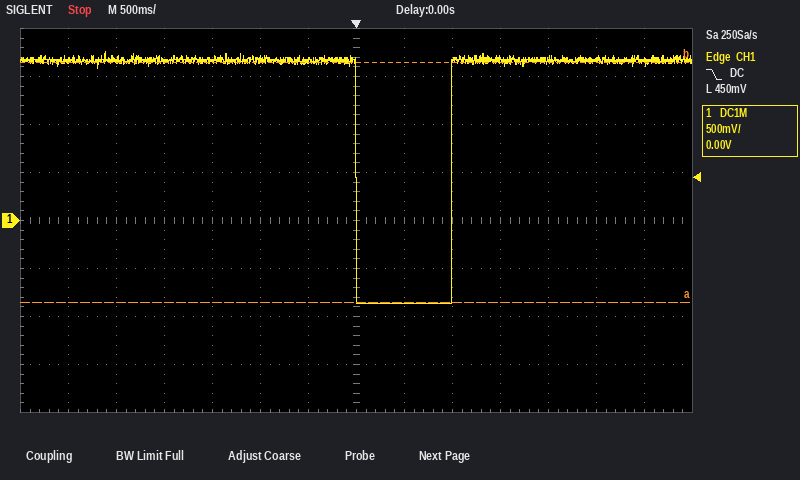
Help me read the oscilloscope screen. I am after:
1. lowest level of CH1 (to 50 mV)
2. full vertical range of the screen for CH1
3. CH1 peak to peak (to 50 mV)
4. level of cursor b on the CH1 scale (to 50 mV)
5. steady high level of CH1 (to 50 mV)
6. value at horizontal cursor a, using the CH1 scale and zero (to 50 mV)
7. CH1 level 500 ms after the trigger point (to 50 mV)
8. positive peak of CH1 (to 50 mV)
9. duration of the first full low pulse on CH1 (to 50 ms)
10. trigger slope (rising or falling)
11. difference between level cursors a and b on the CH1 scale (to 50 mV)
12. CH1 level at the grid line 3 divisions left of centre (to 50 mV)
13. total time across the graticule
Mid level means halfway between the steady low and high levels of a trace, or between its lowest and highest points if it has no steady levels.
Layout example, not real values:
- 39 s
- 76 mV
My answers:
- -850 mV
- 4 V
- 2.60 V
- 1.65 V
- 1.65 V
- -850 mV
- -850 mV
- 1.75 V
- 1.00 s
- falling
- 2.50 V
- 1.65 V
- 7 s
